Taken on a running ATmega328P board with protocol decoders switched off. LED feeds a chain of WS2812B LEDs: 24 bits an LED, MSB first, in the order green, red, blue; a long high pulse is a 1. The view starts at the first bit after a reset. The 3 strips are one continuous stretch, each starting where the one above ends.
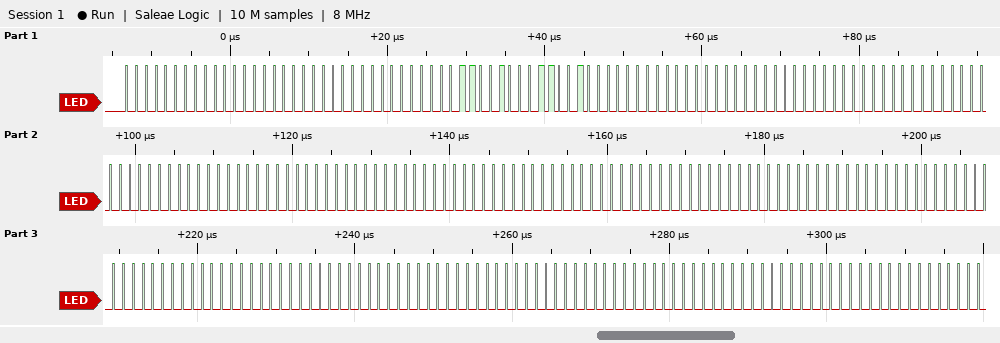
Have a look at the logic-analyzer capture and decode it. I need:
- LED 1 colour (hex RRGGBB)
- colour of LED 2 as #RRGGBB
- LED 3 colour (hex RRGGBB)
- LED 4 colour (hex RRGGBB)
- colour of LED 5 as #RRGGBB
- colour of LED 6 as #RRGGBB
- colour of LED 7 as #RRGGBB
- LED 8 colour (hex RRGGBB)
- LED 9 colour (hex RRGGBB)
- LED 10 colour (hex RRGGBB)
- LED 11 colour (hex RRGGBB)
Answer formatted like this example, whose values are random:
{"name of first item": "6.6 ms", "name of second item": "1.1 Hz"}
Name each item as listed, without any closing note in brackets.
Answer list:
{"LED 1 colour": "#000000", "colour of LED 2 as #RRGGBB": "#320032", "LED 3 colour": "#000000", "LED 4 colour": "#000000", "colour of LED 5 as #RRGGBB": "#000000", "colour of LED 6 as #RRGGBB": "#000000", "colour of LED 7 as #RRGGBB": "#000000", "LED 8 colour": "#000000", "LED 9 colour": "#000000", "LED 10 colour": "#000000", "LED 11 colour": "#000000"}
